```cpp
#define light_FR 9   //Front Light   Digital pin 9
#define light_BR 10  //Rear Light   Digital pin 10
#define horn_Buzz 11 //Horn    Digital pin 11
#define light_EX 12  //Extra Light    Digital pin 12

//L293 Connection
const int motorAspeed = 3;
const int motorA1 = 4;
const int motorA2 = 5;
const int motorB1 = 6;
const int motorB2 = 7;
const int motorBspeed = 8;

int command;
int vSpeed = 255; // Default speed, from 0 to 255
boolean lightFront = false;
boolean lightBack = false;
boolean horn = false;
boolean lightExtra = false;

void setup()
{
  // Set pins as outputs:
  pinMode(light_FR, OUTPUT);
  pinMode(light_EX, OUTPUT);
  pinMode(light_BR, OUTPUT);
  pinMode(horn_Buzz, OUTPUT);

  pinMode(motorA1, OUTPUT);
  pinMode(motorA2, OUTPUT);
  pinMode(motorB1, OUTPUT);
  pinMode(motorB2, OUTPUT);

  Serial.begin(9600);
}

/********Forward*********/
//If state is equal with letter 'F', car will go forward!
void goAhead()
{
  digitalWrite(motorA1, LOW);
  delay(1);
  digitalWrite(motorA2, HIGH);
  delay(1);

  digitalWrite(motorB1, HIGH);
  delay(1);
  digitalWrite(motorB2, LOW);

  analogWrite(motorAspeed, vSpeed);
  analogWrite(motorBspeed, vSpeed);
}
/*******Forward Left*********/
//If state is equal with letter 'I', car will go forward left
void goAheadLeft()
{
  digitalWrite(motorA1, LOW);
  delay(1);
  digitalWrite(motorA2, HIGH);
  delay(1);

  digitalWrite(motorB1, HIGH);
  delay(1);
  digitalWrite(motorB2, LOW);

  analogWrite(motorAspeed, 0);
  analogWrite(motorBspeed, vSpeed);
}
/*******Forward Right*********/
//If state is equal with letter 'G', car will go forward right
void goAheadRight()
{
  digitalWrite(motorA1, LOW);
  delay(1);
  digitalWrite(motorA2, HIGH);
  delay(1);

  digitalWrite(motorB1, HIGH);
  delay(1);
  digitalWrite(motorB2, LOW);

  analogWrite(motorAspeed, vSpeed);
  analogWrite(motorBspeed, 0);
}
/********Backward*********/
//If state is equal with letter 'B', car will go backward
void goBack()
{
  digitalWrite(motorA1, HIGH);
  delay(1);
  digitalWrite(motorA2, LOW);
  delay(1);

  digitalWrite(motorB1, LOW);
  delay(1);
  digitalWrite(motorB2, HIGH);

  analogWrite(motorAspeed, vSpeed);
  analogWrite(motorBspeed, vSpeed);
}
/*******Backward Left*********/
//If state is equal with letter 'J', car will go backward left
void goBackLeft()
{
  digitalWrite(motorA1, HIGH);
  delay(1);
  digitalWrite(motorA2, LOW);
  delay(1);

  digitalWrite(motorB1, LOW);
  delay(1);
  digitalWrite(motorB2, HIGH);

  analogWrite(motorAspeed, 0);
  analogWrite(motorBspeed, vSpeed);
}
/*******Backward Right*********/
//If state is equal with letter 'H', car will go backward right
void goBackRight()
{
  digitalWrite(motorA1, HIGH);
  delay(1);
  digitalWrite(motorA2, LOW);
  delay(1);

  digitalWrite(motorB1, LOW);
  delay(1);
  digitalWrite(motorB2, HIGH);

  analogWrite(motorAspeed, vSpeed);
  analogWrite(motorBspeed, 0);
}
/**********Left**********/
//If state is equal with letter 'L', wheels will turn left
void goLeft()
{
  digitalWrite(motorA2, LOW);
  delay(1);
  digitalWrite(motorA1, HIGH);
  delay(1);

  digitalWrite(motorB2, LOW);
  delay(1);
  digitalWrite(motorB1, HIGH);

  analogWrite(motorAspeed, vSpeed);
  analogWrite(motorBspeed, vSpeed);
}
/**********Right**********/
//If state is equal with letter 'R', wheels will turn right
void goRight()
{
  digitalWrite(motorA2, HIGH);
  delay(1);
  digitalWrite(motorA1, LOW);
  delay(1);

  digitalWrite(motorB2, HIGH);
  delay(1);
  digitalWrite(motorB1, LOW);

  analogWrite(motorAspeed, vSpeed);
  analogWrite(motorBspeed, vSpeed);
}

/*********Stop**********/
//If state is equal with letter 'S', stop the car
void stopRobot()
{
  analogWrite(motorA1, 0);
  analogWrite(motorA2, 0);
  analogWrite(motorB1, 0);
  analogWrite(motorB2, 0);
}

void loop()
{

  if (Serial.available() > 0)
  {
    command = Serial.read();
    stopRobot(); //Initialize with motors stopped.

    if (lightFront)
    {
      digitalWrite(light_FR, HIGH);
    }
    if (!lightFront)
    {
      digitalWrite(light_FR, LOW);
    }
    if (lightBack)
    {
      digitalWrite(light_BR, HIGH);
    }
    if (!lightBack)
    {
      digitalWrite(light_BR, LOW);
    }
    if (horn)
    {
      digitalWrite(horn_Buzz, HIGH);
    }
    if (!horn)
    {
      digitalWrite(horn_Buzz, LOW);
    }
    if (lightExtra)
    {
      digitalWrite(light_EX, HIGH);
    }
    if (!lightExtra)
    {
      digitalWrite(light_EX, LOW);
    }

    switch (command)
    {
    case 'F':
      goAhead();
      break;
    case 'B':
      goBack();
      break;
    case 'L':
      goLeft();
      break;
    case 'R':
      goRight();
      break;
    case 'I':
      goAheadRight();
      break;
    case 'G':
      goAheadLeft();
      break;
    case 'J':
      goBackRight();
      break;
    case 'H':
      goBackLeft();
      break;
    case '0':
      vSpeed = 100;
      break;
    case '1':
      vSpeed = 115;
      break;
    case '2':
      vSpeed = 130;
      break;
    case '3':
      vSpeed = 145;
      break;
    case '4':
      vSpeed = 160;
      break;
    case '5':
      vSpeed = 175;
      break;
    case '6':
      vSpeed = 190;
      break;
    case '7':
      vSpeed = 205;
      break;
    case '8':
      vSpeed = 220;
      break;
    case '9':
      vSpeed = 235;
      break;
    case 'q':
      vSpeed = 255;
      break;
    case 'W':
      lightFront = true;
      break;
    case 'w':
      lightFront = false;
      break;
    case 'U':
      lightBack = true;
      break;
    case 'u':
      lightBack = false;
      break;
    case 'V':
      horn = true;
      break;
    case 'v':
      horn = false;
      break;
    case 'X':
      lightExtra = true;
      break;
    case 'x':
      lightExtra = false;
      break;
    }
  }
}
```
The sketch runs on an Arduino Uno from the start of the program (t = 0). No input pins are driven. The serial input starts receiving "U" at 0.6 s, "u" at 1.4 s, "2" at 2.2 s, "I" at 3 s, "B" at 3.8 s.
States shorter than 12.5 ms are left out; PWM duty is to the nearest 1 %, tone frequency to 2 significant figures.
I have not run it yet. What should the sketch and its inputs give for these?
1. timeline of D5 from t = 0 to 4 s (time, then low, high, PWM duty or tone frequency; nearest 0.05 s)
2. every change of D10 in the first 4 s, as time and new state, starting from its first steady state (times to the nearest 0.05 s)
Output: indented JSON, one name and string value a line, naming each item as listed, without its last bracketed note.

{
  "timeline of D5 from t = 0 to 4 s": "0 s low; 3 s high; 3.8 s low",
  "every change of D10 in the first 4 s, as time and new state, starting from its first steady state": "0 s low; 1.4 s high; 2.2 s low"
}
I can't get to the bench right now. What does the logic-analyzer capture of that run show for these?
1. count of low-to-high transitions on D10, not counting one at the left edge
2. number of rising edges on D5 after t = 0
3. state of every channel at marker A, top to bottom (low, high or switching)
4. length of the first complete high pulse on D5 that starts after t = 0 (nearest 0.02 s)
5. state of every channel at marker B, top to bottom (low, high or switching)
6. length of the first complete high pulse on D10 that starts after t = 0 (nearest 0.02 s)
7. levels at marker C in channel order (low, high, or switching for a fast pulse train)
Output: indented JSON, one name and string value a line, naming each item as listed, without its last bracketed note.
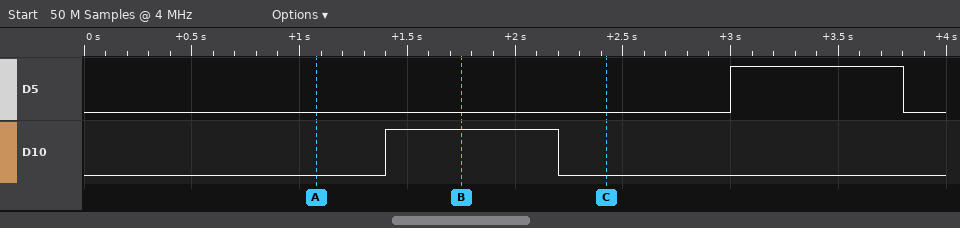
{
  "count of low-to-high transitions on D10, not counting one at the left edge": "1",
  "number of rising edges on D5 after t = 0": "1",
  "state of every channel at marker A, top to bottom": "D5 low, D10 low",
  "length of the first complete high pulse on D5 that starts after t = 0": "0.80 s",
  "state of every channel at marker B, top to bottom": "D5 low, D10 high",
  "length of the first complete high pulse on D10 that starts after t = 0": "0.80 s",
  "levels at marker C in channel order": "D5 low, D10 low"
}
